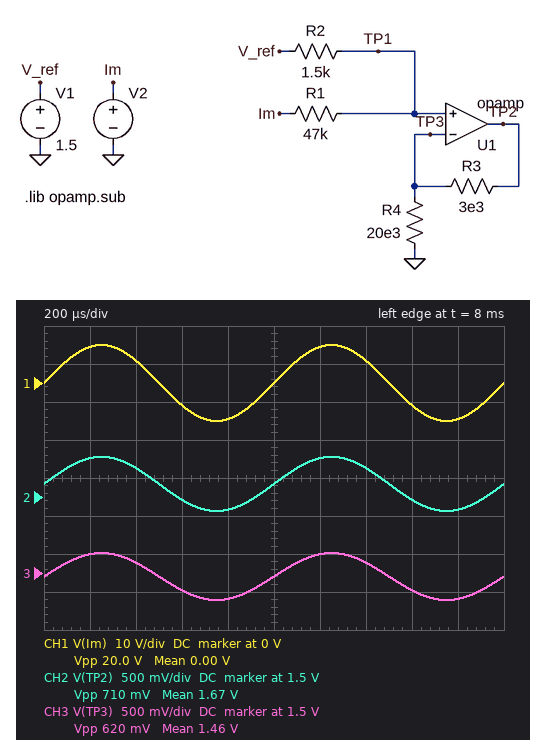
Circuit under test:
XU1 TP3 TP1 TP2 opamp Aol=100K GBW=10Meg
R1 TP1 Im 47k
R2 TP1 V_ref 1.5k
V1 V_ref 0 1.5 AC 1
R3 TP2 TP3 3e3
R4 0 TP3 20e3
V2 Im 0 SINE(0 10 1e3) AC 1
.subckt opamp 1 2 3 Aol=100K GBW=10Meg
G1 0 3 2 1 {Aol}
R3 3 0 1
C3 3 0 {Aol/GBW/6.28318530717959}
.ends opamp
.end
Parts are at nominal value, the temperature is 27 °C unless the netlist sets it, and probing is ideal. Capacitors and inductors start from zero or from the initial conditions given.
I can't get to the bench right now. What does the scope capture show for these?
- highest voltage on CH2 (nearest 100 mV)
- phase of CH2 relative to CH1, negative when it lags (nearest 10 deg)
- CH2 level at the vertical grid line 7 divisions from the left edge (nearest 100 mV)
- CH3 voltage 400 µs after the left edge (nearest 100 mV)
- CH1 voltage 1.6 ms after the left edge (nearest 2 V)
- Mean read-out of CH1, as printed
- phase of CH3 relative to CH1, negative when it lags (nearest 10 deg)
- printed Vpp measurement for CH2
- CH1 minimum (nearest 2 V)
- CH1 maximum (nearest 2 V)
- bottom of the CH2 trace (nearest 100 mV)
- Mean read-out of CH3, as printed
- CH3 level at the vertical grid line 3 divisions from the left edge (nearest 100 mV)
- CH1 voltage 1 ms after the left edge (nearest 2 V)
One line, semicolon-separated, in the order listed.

2.0 V; 0 deg; 1.9 V; 1.6 V; -6 V; 0.00 V; 0 deg; 710 mV; -10 V; 10 V; 1.3 V; 1.46 V; 1.3 V; 0 V
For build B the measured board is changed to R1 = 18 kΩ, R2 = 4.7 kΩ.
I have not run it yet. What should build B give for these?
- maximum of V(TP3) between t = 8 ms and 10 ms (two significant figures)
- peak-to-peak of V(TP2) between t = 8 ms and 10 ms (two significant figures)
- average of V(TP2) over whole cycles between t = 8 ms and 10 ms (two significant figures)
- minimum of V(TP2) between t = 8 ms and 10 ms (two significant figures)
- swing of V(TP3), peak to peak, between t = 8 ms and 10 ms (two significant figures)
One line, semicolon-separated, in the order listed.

3.3 V; 4.8 V; 1.4 V; -1.0 V; 4.1 V
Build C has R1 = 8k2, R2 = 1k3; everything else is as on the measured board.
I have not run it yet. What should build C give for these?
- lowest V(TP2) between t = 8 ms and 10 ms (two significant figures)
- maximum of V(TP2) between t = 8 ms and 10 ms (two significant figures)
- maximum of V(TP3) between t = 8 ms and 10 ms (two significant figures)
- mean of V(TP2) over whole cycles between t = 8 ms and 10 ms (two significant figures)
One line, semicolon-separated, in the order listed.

-85 mV; 3.1 V; 2.7 V; 1.5 V
